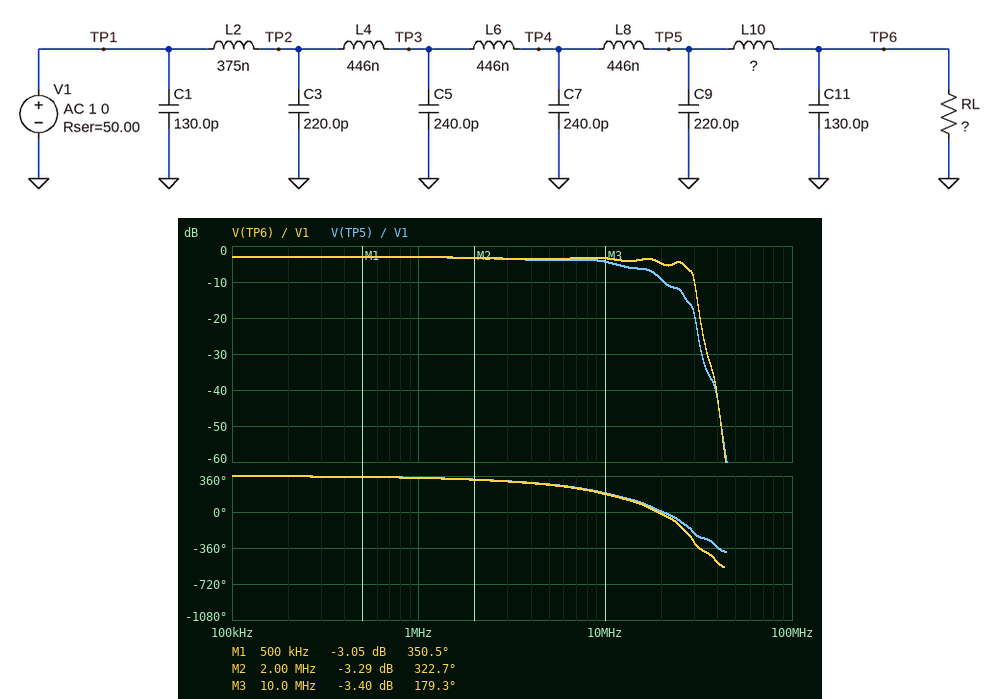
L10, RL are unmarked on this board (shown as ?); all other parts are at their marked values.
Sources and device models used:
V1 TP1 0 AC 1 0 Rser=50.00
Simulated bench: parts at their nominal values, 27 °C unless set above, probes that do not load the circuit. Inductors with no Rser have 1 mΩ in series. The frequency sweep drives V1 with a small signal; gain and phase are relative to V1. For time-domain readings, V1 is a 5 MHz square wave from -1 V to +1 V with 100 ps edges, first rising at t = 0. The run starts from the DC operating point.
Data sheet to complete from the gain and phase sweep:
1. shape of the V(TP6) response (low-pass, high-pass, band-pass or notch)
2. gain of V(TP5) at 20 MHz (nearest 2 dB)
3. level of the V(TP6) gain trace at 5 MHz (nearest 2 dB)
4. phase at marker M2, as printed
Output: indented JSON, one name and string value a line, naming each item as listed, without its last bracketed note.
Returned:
{
  "shape of the V(TP6) response": "low-pass",
  "gain of V(TP5) at 20 MHz": "-10 dB",
  "level of the V(TP6) gain trace at 5 MHz": "-4 dB",
  "phase at marker M2, as printed": "322.7 deg"
}
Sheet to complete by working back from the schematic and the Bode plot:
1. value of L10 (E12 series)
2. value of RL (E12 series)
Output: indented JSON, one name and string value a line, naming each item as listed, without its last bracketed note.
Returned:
{
  "value of L10": "220 nH",
  "value of RL": "120 Ω"
}
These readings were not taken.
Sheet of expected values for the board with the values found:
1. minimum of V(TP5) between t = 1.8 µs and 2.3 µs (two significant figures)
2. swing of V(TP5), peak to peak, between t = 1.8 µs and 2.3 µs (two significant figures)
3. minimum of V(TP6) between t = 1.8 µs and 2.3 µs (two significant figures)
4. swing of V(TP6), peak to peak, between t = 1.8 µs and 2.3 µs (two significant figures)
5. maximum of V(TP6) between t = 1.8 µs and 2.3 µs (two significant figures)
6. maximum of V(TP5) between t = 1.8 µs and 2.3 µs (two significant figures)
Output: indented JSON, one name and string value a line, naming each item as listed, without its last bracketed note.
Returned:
{
  "minimum of V(TP5) between t = 1.8 µs and 2.3 µs": "-710 mV",
  "swing of V(TP5), peak to peak, between t = 1.8 µs and 2.3 µs": "1.4 V",
  "minimum of V(TP6) between t = 1.8 µs and 2.3 µs": "-880 mV",
  "swing of V(TP6), peak to peak, between t = 1.8 µs and 2.3 µs": "1.8 V",
  "maximum of V(TP6) between t = 1.8 µs and 2.3 µs": "880 mV",
  "maximum of V(TP5) between t = 1.8 µs and 2.3 µs": "710 mV"
}
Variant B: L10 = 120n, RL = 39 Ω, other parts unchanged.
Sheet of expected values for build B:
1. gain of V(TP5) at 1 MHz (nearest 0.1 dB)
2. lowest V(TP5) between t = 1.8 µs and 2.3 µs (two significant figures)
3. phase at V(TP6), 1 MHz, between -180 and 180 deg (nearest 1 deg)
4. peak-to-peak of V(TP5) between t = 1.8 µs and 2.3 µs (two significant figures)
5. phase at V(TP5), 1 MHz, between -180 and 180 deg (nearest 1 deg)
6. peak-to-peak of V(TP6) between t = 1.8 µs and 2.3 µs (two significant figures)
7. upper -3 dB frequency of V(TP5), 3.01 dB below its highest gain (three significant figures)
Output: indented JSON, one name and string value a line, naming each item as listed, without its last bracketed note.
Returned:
{
  "gain of V(TP5) at 1 MHz": "-7.2 dB",
  "lowest V(TP5) between t = 1.8 µs and 2.3 µs": "-540 mV",
  "phase at V(TP6), 1 MHz, between -180 and 180 deg": "-17 deg",
  "peak-to-peak of V(TP5) between t = 1.8 µs and 2.3 µs": "1.1 V",
  "phase at V(TP5), 1 MHz, between -180 and 180 deg": "-16 deg",
  "peak-to-peak of V(TP6) between t = 1.8 µs and 2.3 µs": "1.2 V",
  "upper -3 dB frequency of V(TP5), 3.01 dB below its highest gain": "20.7 MHz"
}
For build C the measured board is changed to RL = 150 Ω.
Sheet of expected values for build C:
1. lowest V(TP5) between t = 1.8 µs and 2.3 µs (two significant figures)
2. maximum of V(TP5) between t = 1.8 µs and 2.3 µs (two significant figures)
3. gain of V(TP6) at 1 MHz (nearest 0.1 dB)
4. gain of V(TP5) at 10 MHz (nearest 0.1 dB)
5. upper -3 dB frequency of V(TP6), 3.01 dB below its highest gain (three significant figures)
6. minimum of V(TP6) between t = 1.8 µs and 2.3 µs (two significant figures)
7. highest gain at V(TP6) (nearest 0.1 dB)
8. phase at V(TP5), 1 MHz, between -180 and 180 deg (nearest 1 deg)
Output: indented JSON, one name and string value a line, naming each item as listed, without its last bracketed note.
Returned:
{
  "lowest V(TP5) between t = 1.8 µs and 2.3 µs": "-750 mV",
  "maximum of V(TP5) between t = 1.8 µs and 2.3 µs": "750 mV",
  "gain of V(TP6) at 1 MHz": "-2.6 dB",
  "gain of V(TP5) at 10 MHz": "-3.9 dB",
  "upper -3 dB frequency of V(TP6), 3.01 dB below its highest gain": "26.9 MHz",
  "minimum of V(TP6) between t = 1.8 µs and 2.3 µs": "-920 mV",
  "highest gain at V(TP6)": "-2.5 dB",
  "phase at V(TP5), 1 MHz, between -180 and 180 deg": "-19 deg"
}
